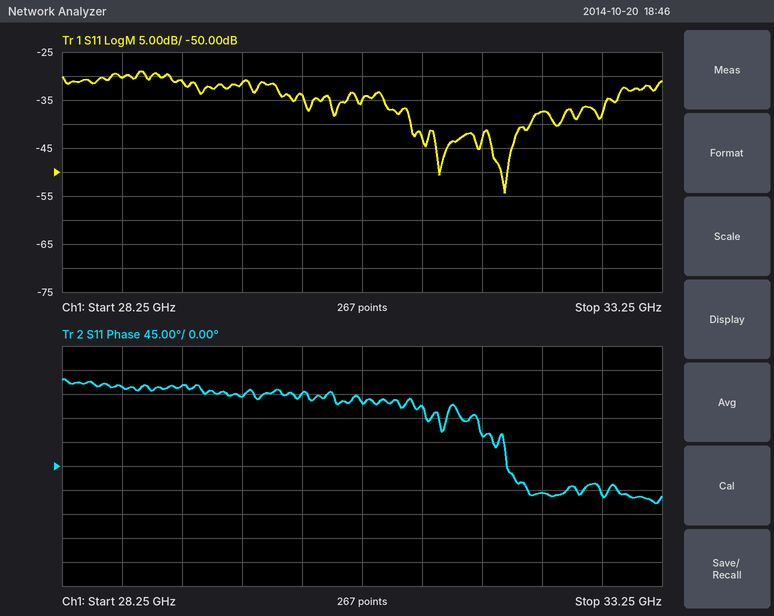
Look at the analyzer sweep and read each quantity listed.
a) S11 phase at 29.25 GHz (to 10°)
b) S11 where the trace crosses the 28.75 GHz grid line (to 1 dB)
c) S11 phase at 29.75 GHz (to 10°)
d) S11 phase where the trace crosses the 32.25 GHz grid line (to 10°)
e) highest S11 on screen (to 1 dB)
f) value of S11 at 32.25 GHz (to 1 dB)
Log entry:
150°
-30 dB
130°
-50°
-29 dB
-37 dB
